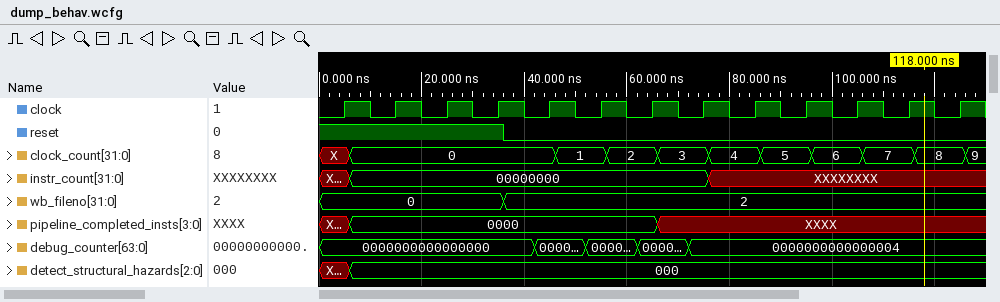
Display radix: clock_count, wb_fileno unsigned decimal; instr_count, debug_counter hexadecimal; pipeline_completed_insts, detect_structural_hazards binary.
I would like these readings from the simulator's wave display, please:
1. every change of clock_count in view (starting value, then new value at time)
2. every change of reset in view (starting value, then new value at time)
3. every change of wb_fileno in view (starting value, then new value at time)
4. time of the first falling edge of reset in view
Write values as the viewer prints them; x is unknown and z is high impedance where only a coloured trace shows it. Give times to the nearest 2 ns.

X, 0 at 6 ns, 1 at 46 ns, 2 at 56 ns, 3 at 66 ns, 4 at 76 ns, 5 at 86 ns, 6 at 96 ns, 7 at 106 ns, 8 at 116 ns, 9 at 126 ns
1, 0 at 36 ns
0, 2 at 36 ns
36 ns
